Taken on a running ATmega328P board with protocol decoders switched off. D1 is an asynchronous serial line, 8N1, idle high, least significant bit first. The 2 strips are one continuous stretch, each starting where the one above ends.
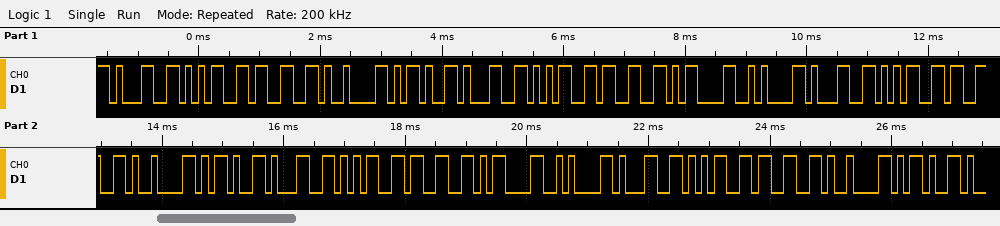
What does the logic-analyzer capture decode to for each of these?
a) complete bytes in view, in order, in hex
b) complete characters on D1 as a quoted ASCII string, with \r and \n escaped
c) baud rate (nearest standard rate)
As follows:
31 35 33 09 2D 31 35 33 0D 0A 31 35 33 09 2D 31 35 33 0D 0A 31 35 33 09 2D
"153\t-153\r\n153\t-153\r\n153\t-"
9600 baud
